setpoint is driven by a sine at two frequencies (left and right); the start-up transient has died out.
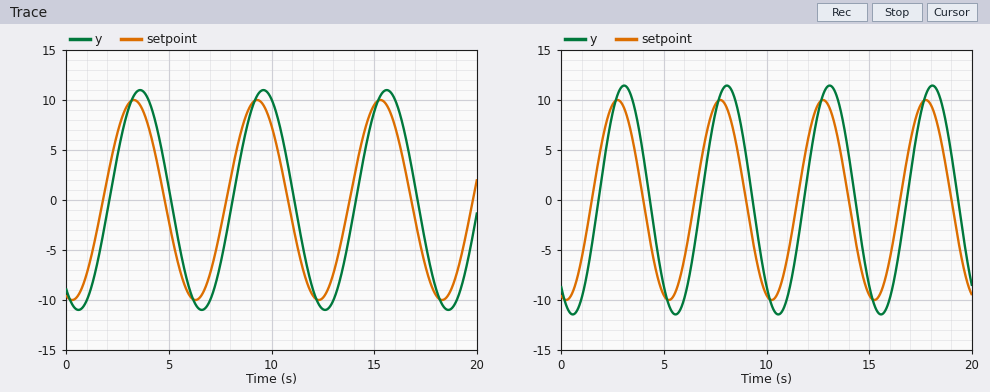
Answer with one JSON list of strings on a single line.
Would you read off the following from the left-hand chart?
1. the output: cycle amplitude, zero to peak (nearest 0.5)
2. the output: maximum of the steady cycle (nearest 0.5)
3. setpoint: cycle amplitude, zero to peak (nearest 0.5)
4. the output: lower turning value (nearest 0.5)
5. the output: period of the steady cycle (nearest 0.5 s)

["11.0", "11.0", "10.0", "-11.0", "6.0 s"]
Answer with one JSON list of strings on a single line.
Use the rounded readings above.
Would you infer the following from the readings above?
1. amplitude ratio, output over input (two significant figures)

["1.1"]
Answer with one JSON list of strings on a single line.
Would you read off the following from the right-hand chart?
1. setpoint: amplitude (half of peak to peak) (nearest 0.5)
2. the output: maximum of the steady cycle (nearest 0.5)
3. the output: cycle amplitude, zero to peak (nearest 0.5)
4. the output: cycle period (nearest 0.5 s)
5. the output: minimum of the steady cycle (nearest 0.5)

["10.0", "11.5", "11.5", "5.0 s", "-11.5"]
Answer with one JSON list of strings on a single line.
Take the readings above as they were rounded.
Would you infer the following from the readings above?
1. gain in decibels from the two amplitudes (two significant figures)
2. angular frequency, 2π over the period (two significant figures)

["1.2 dB", "1.3 rad/s"]
